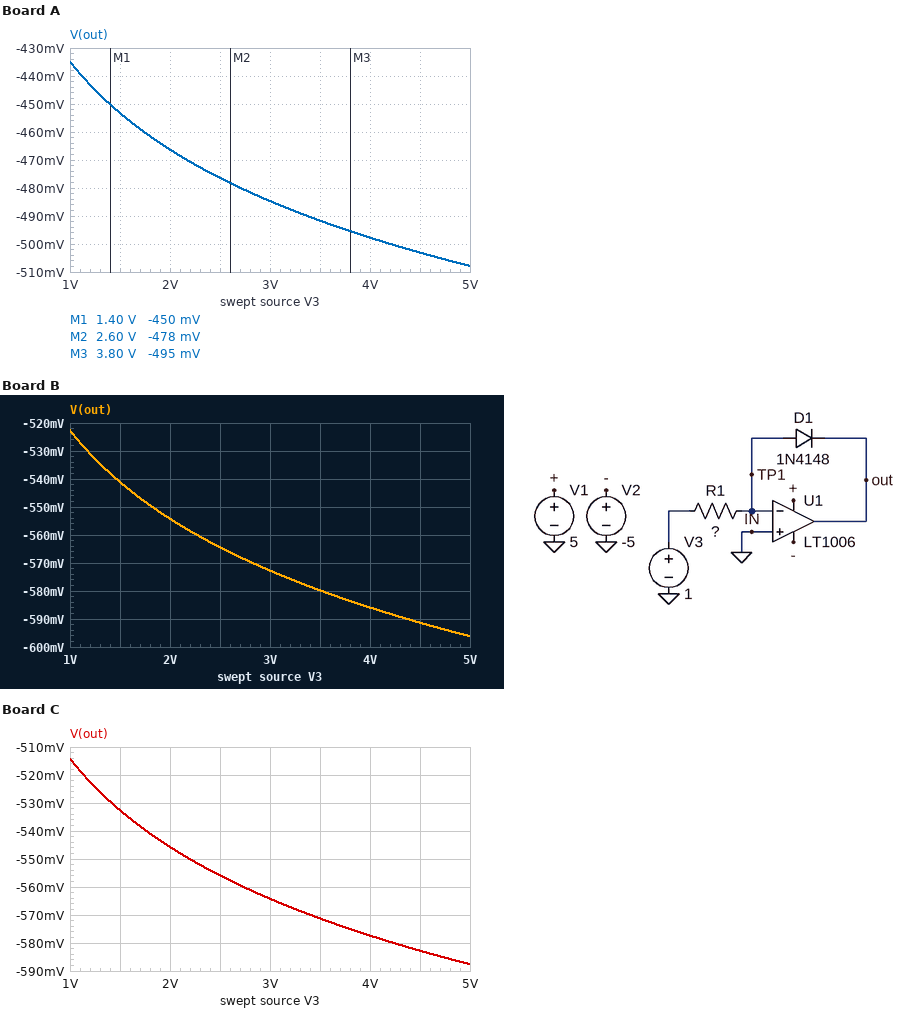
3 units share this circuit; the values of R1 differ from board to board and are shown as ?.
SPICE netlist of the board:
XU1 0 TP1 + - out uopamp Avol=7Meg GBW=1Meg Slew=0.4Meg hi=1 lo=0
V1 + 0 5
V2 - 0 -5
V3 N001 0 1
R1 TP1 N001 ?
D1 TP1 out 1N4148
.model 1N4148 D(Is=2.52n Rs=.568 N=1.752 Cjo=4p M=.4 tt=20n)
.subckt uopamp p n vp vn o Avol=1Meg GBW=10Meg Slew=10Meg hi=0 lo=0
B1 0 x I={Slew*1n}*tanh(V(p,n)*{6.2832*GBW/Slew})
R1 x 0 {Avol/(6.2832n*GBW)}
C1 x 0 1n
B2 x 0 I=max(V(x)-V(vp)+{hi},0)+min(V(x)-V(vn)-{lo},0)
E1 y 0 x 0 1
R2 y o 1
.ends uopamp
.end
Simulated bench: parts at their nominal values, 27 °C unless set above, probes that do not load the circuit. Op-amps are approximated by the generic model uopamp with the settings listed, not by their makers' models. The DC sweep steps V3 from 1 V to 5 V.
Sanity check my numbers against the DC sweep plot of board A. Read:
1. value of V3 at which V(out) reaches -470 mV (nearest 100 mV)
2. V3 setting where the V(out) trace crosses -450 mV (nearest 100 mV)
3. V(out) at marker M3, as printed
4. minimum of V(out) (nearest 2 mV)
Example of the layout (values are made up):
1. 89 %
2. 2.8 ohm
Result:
1. 2.2 V
2. 1.4 V
3. -495 mV
4. -508 mV
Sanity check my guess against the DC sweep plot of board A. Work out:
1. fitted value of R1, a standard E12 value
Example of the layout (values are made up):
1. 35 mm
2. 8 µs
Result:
1. 27 kΩ
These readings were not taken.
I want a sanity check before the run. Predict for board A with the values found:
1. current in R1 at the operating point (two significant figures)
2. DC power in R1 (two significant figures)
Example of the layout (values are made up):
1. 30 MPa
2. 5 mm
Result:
1. 37 µA
2. 37 µW
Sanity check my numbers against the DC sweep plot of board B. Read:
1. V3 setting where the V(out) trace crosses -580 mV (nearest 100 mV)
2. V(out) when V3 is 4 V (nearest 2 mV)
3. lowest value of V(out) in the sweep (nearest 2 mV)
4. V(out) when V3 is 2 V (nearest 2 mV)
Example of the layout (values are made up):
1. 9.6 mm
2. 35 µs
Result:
1. 3.5 V
2. -586 mV
3. -596 mV
4. -554 mV
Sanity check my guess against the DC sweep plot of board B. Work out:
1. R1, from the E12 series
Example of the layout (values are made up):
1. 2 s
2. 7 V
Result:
1. 3.9 kΩ
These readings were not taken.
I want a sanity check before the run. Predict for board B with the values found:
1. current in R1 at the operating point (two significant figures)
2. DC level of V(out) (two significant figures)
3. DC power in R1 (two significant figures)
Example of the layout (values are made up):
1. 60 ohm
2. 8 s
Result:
1. 260 µA
2. -520 mV
3. 260 µW
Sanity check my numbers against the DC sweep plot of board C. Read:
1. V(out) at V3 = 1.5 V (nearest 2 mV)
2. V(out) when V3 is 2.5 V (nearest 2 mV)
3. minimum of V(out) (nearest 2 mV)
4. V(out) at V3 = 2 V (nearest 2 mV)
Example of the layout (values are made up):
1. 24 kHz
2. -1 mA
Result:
1. -532 mV
2. -556 mV
3. -588 mV
4. -546 mV
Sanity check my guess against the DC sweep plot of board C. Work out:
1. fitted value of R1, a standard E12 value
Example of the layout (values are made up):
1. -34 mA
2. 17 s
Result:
1. 4.7 kΩ
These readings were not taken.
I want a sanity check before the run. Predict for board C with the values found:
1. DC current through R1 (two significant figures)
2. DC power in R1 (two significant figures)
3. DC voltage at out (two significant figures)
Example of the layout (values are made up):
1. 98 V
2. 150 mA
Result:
1. 210 µA
2. 210 µW
3. -510 mV
